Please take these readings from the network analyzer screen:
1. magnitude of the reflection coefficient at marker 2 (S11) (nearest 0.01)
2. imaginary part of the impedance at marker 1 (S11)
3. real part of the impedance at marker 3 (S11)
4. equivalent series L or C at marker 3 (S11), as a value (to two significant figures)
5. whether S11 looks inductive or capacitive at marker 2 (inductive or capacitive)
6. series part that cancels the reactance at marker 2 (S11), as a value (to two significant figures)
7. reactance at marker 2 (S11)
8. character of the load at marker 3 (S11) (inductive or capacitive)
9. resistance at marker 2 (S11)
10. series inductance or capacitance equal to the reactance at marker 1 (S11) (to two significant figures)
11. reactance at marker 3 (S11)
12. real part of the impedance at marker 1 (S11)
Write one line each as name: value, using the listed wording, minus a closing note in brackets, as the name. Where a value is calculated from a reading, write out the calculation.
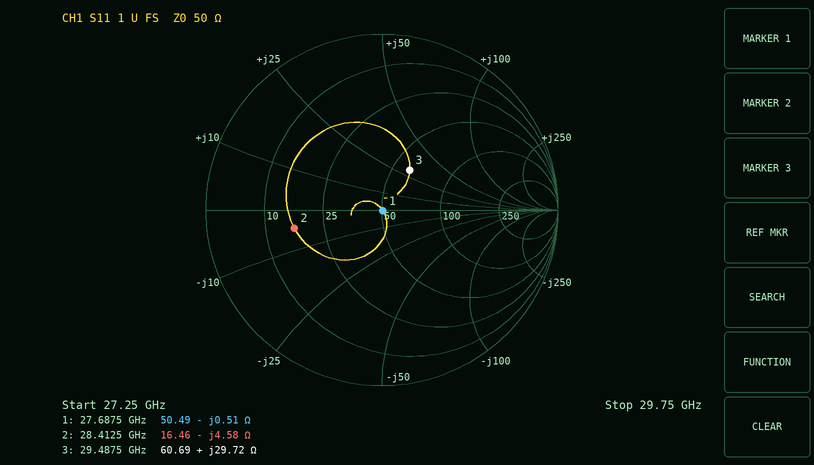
magnitude of the reflection coefficient at marker 2 (S11): 0.51
imaginary part of the impedance at marker 1: -0.51 Ω
real part of the impedance at marker 3: 60.69 Ω
equivalent series L or C at marker 3 (S11), as a value: L = 29.72 Ω/(2π × 29.4875 GHz) ≈ 160 pH
whether S11 looks inductive or capacitive at marker 2: capacitive
series part that cancels the reactance at marker 2 (S11), as a value: L = 4.58 Ω/(2π × 28.4125 GHz) ≈ 26 pH
reactance at marker 2: -4.58 Ω
character of the load at marker 3 (S11): inductive
resistance at marker 2: 16.46 Ω
series inductance or capacitance equal to the reactance at marker 1 (S11): C = 1/(2π × 27.6875 GHz × 0.51 Ω) ≈ 11 pF
reactance at marker 3: +29.72 Ω
real part of the impedance at marker 1: 50.49 Ω
